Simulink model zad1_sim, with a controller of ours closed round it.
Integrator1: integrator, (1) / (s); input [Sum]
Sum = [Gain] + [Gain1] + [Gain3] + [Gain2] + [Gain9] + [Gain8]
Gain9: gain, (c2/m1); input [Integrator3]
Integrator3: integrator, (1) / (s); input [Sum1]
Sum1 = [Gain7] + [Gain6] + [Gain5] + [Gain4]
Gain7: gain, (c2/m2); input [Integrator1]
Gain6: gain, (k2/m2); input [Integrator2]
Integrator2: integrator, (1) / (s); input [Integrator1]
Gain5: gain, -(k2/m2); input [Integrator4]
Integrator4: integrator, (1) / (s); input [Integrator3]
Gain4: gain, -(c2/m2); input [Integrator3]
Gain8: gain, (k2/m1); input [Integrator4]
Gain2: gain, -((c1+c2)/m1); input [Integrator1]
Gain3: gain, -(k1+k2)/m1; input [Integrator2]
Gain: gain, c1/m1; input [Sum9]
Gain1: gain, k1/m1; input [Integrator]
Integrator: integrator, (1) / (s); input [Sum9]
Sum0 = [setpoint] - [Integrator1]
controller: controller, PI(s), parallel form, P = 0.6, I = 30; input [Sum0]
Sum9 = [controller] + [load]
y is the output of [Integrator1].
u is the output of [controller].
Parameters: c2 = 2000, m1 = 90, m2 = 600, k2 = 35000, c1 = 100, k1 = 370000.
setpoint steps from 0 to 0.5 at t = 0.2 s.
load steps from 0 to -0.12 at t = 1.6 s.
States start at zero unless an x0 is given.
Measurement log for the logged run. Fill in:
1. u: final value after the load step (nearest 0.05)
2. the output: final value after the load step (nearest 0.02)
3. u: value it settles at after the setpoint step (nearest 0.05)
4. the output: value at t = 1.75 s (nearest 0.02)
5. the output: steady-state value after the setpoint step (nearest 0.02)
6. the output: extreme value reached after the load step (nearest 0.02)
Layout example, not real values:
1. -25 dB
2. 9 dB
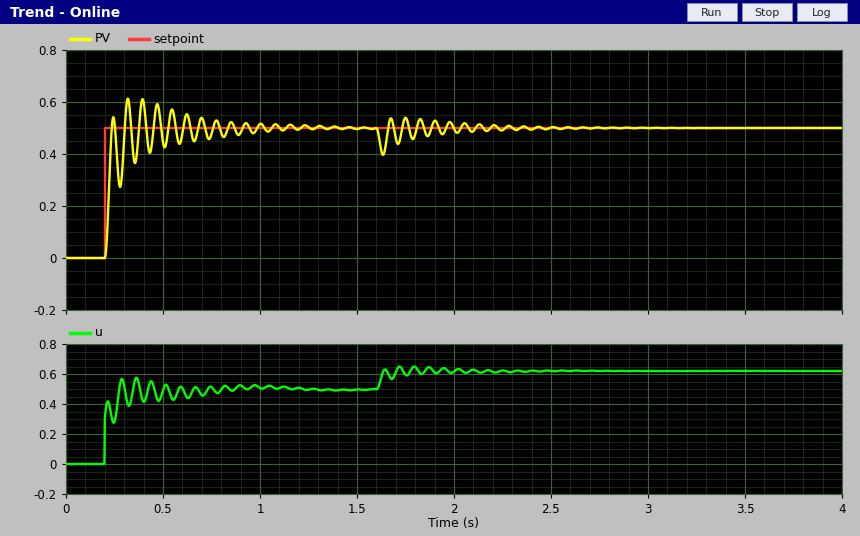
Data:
1. 0.60
2. 0.50
3. 0.50
4. 0.54
5. 0.50
6. 0.40
